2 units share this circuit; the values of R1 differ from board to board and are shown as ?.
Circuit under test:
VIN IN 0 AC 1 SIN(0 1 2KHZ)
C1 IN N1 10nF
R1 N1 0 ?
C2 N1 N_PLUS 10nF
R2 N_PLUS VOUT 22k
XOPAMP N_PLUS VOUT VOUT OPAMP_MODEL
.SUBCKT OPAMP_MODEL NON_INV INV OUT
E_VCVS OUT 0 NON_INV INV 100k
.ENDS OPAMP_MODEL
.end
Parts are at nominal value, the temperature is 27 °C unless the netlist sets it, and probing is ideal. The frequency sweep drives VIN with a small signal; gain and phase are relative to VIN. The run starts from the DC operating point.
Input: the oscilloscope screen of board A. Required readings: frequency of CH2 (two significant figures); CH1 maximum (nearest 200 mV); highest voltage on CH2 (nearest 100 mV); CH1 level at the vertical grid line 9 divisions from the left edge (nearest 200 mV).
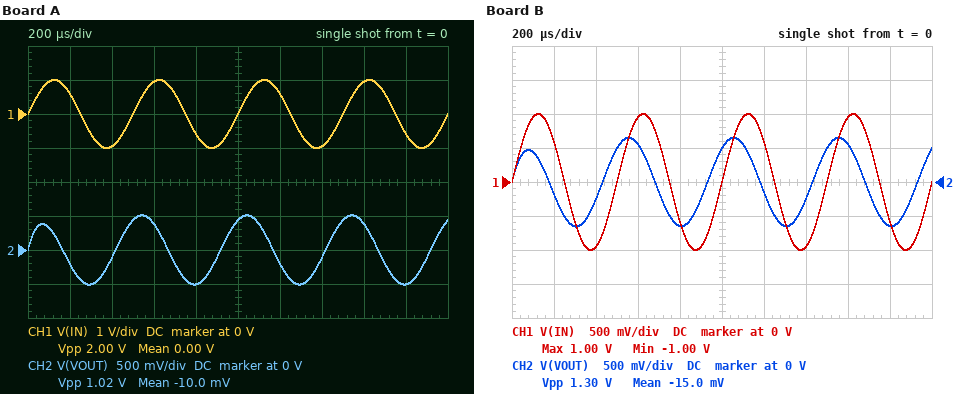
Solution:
2.0 kHz
1.0 V
500 mV
-600 mV
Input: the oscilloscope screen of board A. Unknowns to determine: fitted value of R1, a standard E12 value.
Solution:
4.7 kΩ
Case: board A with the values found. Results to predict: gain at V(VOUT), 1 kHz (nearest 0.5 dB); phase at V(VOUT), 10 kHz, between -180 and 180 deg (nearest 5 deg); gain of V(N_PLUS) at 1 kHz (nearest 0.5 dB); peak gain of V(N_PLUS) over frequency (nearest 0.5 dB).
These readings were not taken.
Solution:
-11.0 dB
20 deg
-11.0 dB
0 dB
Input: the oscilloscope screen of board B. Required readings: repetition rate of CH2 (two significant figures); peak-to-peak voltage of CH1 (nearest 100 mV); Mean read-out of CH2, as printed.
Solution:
2.0 kHz
2.0 V
-15.0 mV
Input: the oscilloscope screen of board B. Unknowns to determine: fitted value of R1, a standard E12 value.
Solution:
6.8 kΩ
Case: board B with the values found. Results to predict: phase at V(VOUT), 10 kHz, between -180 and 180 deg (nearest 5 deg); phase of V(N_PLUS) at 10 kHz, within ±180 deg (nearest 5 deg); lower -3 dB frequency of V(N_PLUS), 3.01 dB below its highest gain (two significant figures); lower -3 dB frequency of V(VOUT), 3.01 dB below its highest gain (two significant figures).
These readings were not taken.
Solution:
15 deg
15 deg
2.3 kHz
2.3 kHz
